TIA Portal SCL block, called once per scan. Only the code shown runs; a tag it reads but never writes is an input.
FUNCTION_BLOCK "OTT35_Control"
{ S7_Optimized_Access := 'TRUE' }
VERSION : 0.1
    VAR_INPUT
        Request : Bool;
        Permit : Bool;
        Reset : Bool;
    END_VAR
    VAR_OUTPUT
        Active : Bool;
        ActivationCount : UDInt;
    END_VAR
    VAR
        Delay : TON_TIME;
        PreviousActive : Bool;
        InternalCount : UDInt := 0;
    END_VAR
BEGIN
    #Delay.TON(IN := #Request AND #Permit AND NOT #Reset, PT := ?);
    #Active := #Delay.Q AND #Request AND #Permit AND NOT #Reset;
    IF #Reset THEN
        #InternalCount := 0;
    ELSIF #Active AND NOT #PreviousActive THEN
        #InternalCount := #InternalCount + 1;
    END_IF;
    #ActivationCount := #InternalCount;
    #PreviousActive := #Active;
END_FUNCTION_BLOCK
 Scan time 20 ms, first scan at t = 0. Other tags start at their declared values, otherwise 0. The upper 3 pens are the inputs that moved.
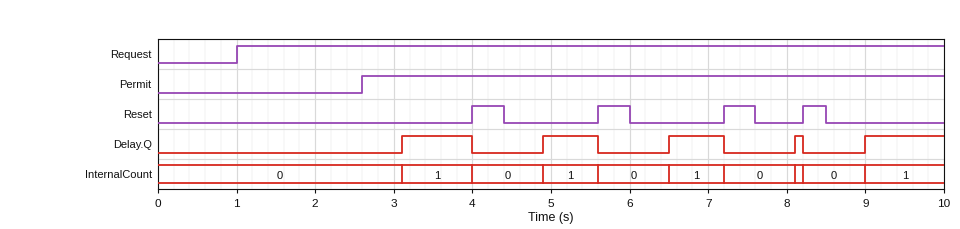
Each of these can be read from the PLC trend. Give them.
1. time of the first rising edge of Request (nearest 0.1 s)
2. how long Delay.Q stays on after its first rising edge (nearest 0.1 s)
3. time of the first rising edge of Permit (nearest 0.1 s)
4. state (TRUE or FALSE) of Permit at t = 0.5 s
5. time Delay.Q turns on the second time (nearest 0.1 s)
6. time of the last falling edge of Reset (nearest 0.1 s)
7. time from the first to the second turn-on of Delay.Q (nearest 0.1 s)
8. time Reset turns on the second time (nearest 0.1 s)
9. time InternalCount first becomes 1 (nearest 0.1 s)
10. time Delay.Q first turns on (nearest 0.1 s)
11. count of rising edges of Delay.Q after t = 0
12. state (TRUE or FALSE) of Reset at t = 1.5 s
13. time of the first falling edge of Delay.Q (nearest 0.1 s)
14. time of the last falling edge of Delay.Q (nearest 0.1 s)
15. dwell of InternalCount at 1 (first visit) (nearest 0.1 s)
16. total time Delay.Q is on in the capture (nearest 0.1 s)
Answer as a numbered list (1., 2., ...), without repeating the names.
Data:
1. 1.0 s
2. 0.9 s
3. 2.6 s
4. FALSE
5. 4.9 s
6. 8.5 s
7. 1.8 s
8. 5.6 s
9. 3.1 s
10. 3.1 s
11. 5
12. FALSE
13. 4.0 s
14. 8.2 s
15. 0.9 s
16. 3.4 s
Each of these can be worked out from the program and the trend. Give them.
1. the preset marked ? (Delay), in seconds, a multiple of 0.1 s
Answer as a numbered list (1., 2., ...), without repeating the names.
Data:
1. 0.5 s
